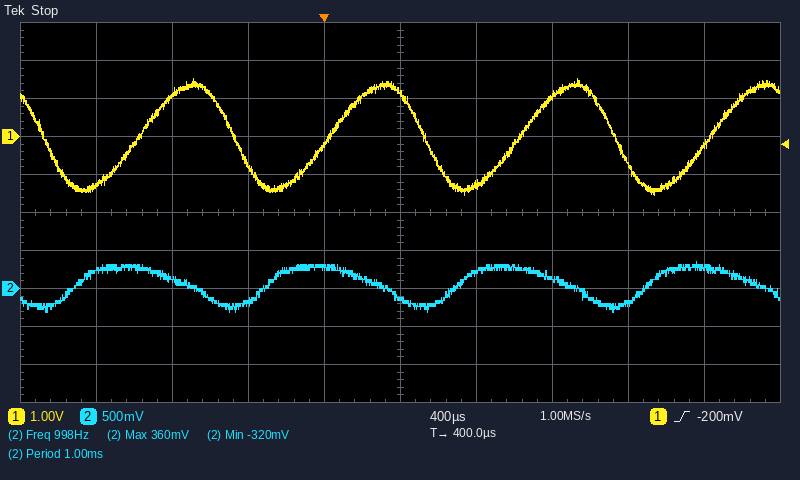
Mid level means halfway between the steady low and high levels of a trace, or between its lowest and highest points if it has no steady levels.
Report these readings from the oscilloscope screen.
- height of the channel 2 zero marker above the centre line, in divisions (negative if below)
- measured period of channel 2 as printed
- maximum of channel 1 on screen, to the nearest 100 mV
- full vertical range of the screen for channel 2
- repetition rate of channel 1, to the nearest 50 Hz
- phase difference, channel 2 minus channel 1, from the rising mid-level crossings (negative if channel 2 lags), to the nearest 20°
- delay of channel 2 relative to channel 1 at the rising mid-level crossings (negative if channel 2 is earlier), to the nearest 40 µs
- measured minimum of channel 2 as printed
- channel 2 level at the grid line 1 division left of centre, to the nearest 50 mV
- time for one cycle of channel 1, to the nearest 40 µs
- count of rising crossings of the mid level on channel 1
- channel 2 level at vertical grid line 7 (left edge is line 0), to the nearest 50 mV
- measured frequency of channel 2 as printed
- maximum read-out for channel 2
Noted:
-2.0 div
1.00 ms
1.5 V
5 V
1.00 kHz
+120°
-320 µs
-320 mV
300 mV
1.00 ms
4
100 mV
998 Hz
360 mV
